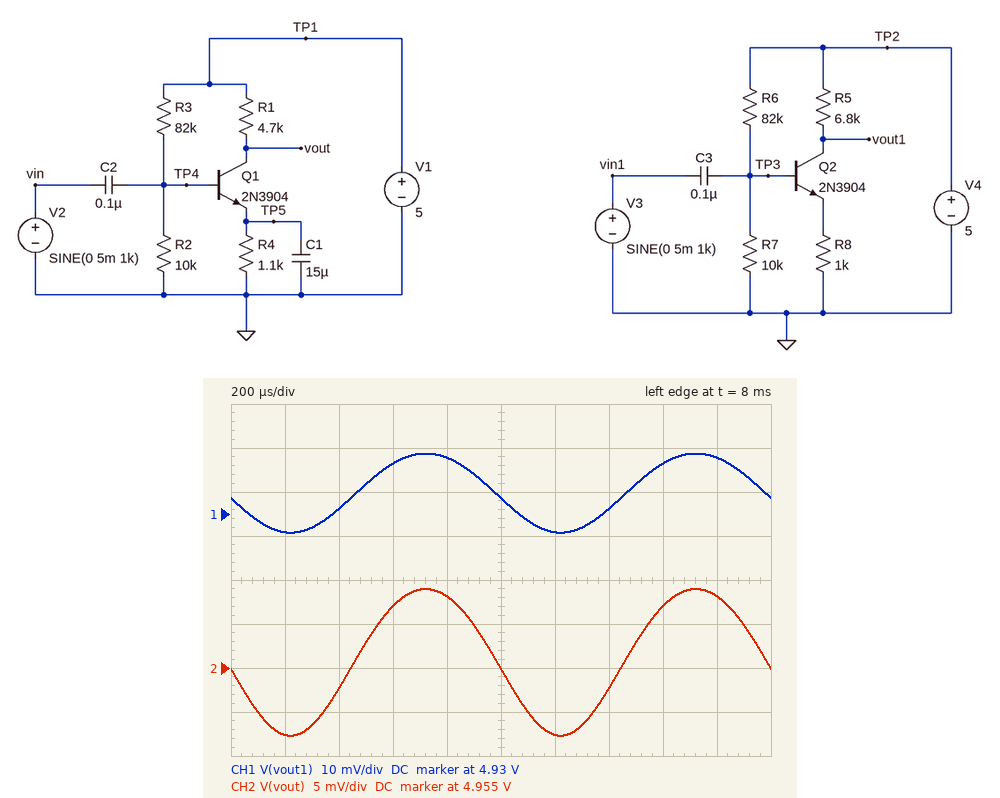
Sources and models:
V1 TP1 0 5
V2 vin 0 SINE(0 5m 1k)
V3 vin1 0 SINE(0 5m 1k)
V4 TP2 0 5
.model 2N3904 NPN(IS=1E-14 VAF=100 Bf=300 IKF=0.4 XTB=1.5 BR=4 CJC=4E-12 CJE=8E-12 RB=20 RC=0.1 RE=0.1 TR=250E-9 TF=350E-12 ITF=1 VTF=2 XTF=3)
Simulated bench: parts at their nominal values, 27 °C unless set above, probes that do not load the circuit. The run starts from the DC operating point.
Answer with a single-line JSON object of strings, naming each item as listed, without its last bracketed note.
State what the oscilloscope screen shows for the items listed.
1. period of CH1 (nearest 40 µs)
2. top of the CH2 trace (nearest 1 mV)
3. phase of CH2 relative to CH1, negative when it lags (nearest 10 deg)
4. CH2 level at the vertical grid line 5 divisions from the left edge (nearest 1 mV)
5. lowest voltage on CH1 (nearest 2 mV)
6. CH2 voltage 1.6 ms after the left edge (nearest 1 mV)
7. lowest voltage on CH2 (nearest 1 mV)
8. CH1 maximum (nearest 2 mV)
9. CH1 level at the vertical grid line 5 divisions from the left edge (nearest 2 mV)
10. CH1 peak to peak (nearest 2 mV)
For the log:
{"period of CH1": "1.00 ms", "top of the CH2 trace": "4.964 V", "phase of CH2 relative to CH1, negative when it lags": "0 deg", "CH2 level at the vertical grid line 5 divisions from the left edge": "4.955 V", "lowest voltage on CH1": "4.926 V", "CH2 voltage 1.6 ms after the left edge": "4.962 V", "lowest voltage on CH2": "4.947 V", "CH1 maximum": "4.944 V", "CH1 level at the vertical grid line 5 divisions from the left edge": "4.934 V", "CH1 peak to peak": "18 mV"}
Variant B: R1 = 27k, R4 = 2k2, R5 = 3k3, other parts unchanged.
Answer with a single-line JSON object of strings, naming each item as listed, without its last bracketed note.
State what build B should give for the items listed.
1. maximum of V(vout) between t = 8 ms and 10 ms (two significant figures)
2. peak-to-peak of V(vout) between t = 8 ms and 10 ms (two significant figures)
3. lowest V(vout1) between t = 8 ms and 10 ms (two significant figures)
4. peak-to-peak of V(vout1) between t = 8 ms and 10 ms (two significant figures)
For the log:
{"maximum of V(vout) between t = 8 ms and 10 ms": "4.8 V", "peak-to-peak of V(vout) between t = 8 ms and 10 ms": "76 mV", "lowest V(vout1) between t = 8 ms and 10 ms": "5.0 V", "peak-to-peak of V(vout1) between t = 8 ms and 10 ms": "8.7 mV"}
